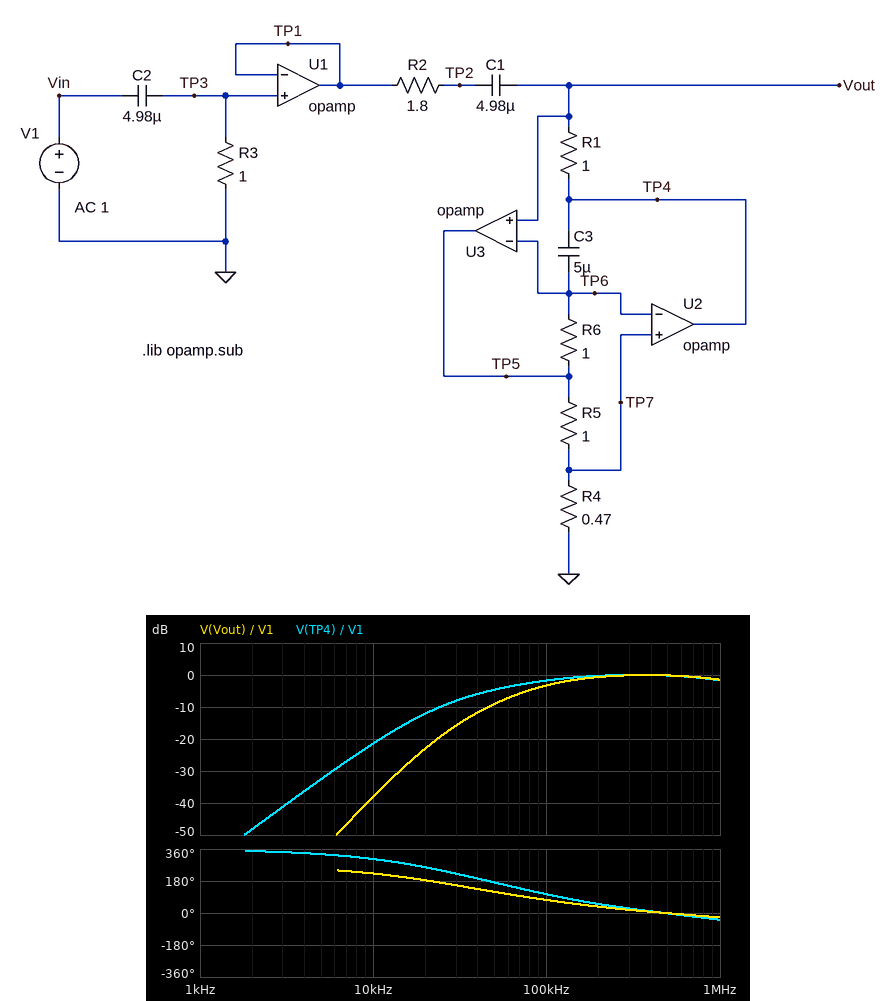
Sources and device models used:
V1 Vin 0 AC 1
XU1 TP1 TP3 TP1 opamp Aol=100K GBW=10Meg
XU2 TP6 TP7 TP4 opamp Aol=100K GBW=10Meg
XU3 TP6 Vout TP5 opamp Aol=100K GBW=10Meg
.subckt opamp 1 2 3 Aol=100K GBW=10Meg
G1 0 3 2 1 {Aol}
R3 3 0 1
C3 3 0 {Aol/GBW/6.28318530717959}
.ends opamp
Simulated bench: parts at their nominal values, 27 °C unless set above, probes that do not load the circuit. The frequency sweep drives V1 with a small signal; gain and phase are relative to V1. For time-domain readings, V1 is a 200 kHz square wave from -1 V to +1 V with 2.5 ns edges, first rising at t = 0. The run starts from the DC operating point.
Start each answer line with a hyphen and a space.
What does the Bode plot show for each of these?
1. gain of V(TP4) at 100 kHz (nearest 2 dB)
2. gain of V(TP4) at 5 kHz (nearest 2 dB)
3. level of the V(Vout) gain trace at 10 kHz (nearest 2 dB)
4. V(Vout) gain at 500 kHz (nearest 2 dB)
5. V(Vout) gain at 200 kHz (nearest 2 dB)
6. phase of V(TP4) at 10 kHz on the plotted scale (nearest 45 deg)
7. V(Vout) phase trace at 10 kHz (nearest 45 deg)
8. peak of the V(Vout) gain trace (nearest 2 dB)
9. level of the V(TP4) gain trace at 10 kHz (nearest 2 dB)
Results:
- -2 dB
- -32 dB
- -38 dB
- 0 dB
- 0 dB
- 315 deg
- 225 deg
- 0 dB
- -22 dB
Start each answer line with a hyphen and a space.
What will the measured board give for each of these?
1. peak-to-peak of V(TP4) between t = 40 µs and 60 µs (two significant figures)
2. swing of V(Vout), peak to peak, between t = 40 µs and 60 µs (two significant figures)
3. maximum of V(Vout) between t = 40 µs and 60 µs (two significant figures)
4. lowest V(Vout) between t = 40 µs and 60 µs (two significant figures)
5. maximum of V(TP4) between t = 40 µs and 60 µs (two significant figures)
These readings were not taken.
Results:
- 3.7 V
- 3.3 V
- 1.6 V
- -1.6 V
- 1.9 V
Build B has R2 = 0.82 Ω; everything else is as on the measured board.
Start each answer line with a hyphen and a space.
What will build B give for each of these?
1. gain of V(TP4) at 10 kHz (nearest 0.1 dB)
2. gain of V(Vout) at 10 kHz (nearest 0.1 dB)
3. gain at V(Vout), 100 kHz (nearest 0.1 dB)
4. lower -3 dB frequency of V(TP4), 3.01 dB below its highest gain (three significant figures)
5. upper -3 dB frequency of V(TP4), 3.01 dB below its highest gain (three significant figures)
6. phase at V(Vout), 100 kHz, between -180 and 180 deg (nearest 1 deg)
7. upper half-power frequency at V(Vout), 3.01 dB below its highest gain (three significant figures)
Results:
- -20.4 dB
- -37.0 dB
- 0.1 dB
- 35.7 kHz
- 759 kHz
- 51 deg
- 2.39 MHz
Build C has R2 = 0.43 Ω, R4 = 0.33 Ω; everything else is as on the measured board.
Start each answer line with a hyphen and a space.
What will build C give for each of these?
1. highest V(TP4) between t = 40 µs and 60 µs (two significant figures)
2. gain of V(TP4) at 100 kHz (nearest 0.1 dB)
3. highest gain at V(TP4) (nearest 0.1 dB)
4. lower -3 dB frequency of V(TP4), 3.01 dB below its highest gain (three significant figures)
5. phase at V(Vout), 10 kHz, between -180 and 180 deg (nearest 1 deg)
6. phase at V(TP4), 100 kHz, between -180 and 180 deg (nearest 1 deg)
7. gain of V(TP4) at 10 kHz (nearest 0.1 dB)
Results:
- 2.0 V
- 4.3 dB
- 7.7 dB
- 43.0 kHz
- -115 deg
- 88 deg
- -20.3 dB
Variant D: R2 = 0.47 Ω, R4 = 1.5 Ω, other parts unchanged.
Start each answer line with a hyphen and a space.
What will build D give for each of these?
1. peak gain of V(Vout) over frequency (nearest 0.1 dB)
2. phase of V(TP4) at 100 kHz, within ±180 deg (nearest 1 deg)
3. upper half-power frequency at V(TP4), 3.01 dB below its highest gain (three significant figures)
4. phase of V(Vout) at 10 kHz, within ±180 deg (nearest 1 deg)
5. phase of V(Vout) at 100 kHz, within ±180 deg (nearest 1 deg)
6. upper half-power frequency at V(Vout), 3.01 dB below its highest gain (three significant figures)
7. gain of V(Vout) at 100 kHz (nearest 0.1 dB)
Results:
- 4.7 dB
- 34 deg
- 36.3 kHz
- -117 deg
- 23 deg
- 40.6 kHz
- 0.1 dB
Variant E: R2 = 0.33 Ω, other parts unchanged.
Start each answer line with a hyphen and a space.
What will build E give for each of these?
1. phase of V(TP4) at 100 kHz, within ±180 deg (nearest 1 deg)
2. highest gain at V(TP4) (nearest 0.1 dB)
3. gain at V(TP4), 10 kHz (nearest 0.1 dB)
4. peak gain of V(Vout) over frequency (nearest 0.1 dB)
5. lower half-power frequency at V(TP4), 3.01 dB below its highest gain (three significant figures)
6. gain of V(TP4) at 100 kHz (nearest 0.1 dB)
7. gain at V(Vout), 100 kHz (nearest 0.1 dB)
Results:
- 64 deg
- 9.9 dB
- -20.1 dB
- 5.3 dB
- 38.8 kHz
- 2.9 dB
- 1.3 dB
